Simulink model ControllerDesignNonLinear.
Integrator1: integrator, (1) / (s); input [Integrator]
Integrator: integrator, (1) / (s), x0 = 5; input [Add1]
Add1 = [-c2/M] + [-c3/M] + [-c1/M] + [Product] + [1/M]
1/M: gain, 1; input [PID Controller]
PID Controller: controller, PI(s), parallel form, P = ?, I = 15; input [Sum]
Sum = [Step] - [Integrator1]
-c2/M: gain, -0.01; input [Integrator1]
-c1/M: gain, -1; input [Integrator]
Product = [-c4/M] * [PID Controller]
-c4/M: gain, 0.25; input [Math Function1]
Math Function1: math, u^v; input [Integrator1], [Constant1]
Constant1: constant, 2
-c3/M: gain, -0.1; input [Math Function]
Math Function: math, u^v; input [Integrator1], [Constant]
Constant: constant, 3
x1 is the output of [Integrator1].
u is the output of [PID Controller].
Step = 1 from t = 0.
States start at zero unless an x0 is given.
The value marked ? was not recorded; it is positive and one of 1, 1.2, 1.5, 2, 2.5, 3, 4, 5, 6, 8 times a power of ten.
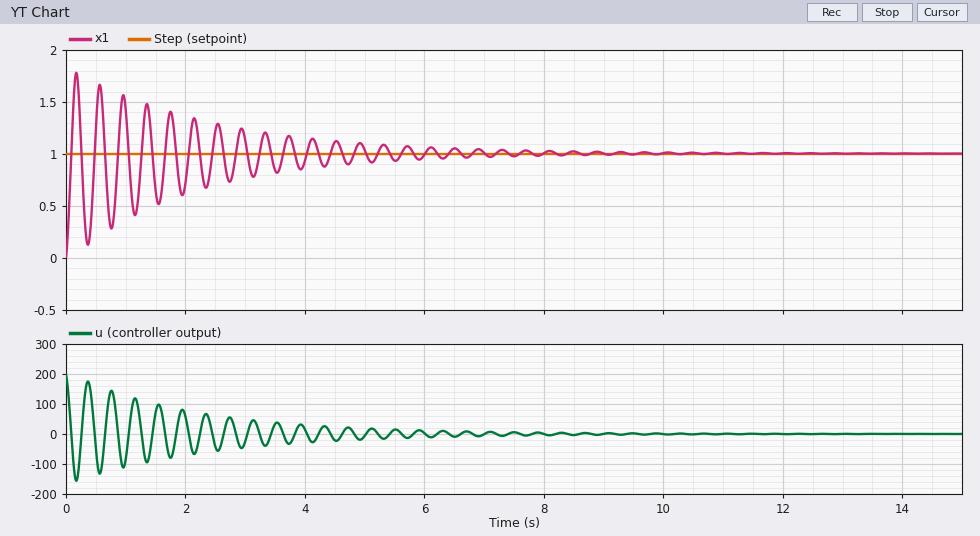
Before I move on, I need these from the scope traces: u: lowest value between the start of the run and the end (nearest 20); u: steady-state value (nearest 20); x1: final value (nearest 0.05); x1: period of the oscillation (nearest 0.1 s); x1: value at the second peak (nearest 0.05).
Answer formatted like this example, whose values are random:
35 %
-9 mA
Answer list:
-160
0
1.00
0.4 s
1.65
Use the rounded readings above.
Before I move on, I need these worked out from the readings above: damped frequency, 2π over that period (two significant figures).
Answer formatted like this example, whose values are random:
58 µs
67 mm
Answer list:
16 rad/s
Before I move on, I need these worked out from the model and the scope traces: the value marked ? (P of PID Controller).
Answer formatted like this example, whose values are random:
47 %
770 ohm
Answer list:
200
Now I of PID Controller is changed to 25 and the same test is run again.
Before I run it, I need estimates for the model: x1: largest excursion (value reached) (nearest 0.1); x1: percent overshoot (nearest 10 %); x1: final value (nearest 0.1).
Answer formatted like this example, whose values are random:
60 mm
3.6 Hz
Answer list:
1.8
80 %
1.0
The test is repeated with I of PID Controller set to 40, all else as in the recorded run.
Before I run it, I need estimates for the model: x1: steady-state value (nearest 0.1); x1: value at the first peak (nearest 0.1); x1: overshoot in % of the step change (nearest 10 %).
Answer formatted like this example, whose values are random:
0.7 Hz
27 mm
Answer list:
1.0
1.8
80 %
